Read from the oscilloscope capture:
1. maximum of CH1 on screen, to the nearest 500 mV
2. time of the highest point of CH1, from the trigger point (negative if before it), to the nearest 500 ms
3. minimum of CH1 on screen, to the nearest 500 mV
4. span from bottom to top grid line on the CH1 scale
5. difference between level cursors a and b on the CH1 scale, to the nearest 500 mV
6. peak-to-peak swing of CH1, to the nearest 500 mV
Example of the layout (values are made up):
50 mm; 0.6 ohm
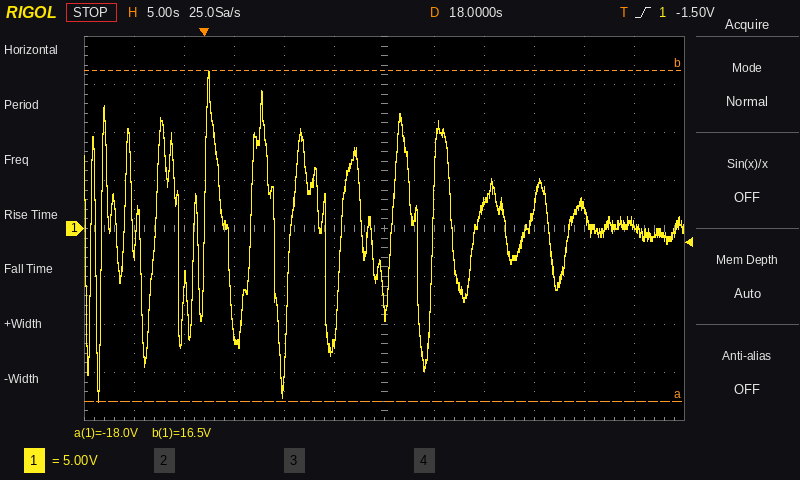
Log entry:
16.5 V; +500 ms; -18.0 V; 40 V; 34.5 V; 34.5 V
